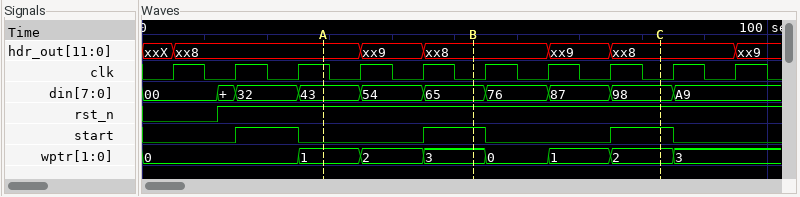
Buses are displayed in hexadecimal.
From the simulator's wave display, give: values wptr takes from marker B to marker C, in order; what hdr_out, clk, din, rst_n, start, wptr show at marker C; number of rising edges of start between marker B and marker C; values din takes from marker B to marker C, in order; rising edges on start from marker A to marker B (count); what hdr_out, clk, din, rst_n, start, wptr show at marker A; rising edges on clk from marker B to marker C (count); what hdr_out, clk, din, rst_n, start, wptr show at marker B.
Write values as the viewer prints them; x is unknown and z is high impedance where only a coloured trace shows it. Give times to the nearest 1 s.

3, 0, 1, 2
hdr_out=xx8, clk=0, din=98, rst_n=1, start=1, wptr=2
1
65, 76, 87, 98
1
hdr_out=xx8, clk=1, din=43, rst_n=1, start=0, wptr=1
3
hdr_out=xx8, clk=0, din=65, rst_n=1, start=1, wptr=3
